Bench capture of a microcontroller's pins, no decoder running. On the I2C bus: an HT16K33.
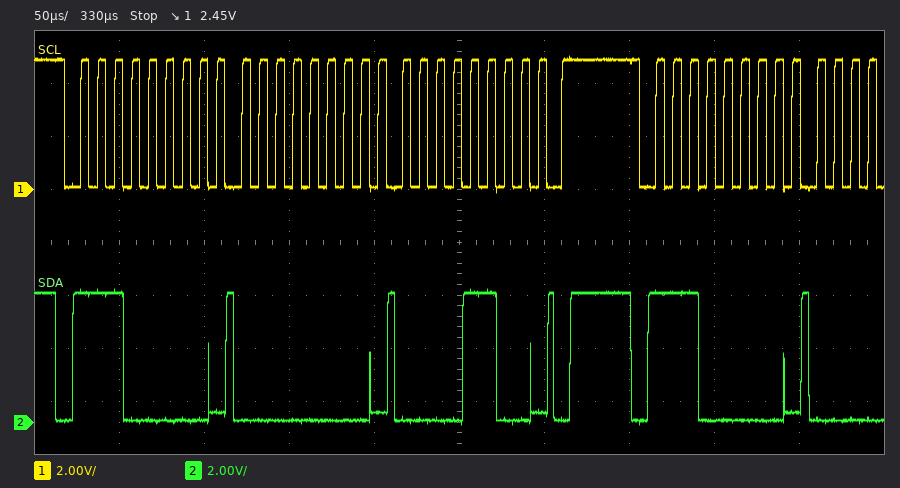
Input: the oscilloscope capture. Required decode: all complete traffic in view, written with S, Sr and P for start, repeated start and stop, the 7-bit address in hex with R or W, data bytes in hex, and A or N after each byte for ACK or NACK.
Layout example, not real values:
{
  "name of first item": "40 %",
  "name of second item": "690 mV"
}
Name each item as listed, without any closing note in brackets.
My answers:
{
  "all complete traffic in view, written with S, Sr and P for start, repeated start and stop, the 7-bit address in hex with R or W, data bytes in hex, and A or N after each byte for ACK or NACK": "S 70W A 00 A 0C A P S 70W A"
}
